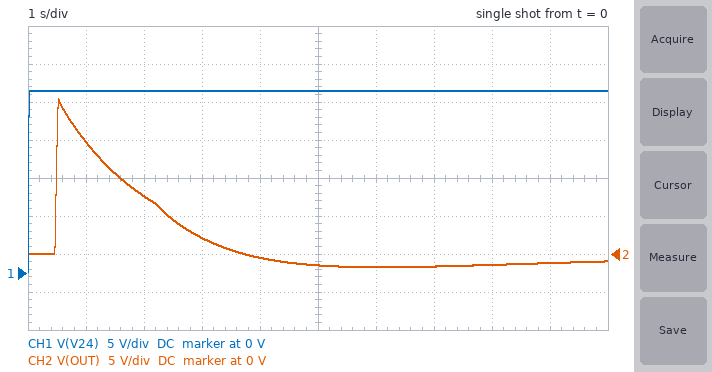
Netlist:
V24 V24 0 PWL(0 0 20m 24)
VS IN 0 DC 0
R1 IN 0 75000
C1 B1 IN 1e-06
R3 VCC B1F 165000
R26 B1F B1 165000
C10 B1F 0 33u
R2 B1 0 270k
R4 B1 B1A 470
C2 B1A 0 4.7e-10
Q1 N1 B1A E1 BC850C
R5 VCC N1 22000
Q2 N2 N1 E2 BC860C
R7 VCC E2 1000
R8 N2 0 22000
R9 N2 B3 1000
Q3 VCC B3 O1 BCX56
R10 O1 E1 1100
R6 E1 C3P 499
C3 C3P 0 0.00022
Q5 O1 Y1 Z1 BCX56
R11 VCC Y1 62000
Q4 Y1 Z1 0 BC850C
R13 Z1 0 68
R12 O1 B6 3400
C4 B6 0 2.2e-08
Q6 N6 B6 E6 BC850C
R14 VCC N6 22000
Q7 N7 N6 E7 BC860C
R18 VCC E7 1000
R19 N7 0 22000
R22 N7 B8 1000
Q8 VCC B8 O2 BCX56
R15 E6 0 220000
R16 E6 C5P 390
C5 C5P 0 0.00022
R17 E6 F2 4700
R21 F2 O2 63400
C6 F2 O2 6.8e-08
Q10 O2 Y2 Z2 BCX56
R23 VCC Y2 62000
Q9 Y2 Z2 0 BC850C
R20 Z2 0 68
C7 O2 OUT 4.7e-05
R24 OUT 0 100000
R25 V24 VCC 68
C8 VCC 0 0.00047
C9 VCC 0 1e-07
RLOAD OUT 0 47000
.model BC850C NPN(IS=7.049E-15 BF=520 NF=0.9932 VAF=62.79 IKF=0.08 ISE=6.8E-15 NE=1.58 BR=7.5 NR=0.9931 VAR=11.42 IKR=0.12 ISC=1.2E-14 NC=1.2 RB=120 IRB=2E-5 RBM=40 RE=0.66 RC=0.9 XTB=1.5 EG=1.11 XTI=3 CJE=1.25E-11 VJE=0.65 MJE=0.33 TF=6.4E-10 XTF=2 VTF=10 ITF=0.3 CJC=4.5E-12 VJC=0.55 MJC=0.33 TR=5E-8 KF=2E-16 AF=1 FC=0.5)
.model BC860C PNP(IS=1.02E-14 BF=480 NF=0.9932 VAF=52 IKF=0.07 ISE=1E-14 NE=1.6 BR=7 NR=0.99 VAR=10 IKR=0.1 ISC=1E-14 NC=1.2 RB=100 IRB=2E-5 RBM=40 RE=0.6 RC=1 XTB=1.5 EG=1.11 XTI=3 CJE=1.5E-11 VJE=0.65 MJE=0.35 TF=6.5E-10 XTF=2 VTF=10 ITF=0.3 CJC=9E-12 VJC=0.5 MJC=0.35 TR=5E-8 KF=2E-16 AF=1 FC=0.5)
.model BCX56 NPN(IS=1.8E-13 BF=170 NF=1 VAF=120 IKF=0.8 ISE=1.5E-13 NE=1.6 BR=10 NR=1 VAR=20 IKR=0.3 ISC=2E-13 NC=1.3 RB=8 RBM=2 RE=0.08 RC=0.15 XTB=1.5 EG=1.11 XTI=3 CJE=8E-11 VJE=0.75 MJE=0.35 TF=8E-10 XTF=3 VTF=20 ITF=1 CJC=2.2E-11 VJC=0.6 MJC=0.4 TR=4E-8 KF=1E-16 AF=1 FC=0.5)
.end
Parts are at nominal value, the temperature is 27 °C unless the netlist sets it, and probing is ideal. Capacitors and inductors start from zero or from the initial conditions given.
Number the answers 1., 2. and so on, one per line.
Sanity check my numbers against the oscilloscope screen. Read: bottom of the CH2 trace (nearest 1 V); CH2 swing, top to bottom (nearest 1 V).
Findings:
1. -2 V
2. 22 V
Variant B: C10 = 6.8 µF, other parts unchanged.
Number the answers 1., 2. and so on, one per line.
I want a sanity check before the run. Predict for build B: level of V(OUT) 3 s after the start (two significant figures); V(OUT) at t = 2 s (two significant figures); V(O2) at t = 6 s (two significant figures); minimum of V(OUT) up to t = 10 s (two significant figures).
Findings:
1. -2.3 V
2. 6.5 V
3. 8.4 V
4. -3.3 V
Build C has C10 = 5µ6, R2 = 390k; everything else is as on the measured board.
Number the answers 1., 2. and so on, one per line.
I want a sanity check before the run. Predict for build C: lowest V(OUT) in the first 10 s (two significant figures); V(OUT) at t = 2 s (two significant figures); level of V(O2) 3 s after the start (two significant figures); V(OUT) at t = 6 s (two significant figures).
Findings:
1. -2.6 V
2. 6.6 V
3. 15 V
4. -1.2 V
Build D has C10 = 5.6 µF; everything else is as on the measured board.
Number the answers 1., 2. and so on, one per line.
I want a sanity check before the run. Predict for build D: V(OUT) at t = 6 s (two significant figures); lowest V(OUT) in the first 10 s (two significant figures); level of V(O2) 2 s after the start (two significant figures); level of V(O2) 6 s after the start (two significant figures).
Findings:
1. -1.0 V
2. -3.1 V
3. 18 V
4. 8.3 V
